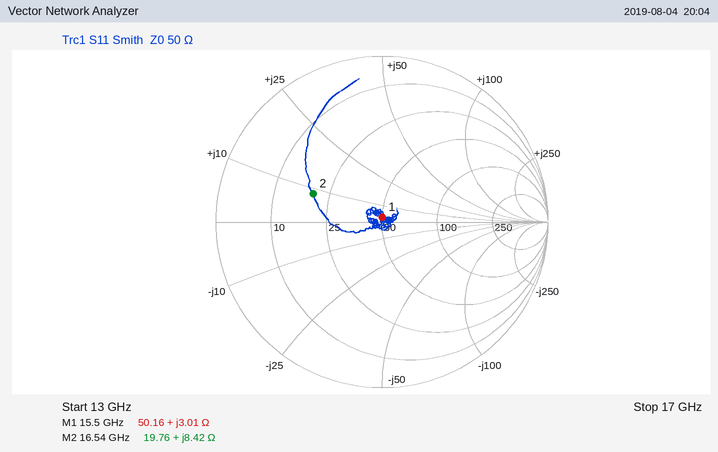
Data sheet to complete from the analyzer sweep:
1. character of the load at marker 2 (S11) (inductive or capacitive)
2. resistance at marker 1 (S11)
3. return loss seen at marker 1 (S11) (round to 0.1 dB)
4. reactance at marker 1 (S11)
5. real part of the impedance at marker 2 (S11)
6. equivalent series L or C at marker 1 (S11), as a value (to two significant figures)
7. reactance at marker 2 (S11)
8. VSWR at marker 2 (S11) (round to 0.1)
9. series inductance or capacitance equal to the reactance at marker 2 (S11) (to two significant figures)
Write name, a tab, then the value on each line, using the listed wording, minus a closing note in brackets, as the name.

character of the load at marker 2 (S11)	inductive
resistance at marker 1	50.16 Ω
return loss seen at marker 1 (S11)	30.4 dB
reactance at marker 1	+3.01 Ω
real part of the impedance at marker 2	19.76 Ω
equivalent series L or C at marker 1 (S11), as a value	31 pH
reactance at marker 2	+8.42 Ω
VSWR at marker 2 (S11)	2.6
series inductance or capacitance equal to the reactance at marker 2 (S11)	81 pH
